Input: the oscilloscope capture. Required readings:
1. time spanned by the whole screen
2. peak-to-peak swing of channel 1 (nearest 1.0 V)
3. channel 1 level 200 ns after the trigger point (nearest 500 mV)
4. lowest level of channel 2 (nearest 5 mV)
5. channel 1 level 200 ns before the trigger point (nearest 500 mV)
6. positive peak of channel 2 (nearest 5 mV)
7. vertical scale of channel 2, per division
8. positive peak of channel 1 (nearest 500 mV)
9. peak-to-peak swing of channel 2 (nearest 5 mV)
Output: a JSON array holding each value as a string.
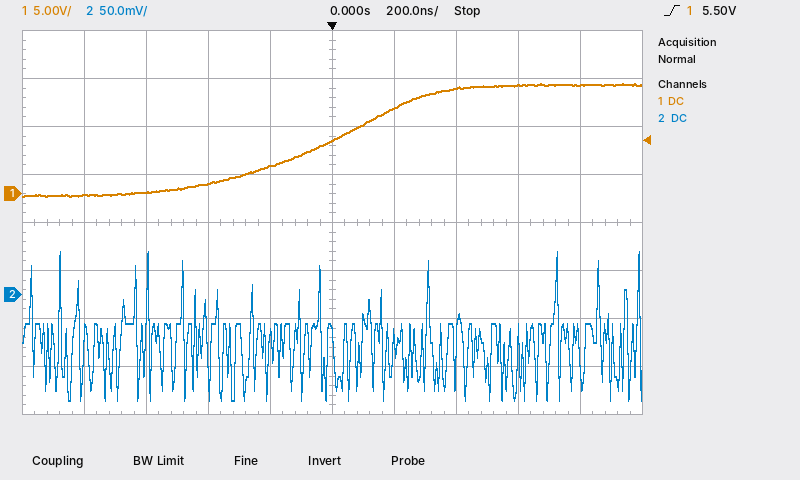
["2 µs", "12.0 V", "9.0 V", "-110 mV", "3.0 V", "45 mV", "50 mV", "11.5 V", "155 mV"]
